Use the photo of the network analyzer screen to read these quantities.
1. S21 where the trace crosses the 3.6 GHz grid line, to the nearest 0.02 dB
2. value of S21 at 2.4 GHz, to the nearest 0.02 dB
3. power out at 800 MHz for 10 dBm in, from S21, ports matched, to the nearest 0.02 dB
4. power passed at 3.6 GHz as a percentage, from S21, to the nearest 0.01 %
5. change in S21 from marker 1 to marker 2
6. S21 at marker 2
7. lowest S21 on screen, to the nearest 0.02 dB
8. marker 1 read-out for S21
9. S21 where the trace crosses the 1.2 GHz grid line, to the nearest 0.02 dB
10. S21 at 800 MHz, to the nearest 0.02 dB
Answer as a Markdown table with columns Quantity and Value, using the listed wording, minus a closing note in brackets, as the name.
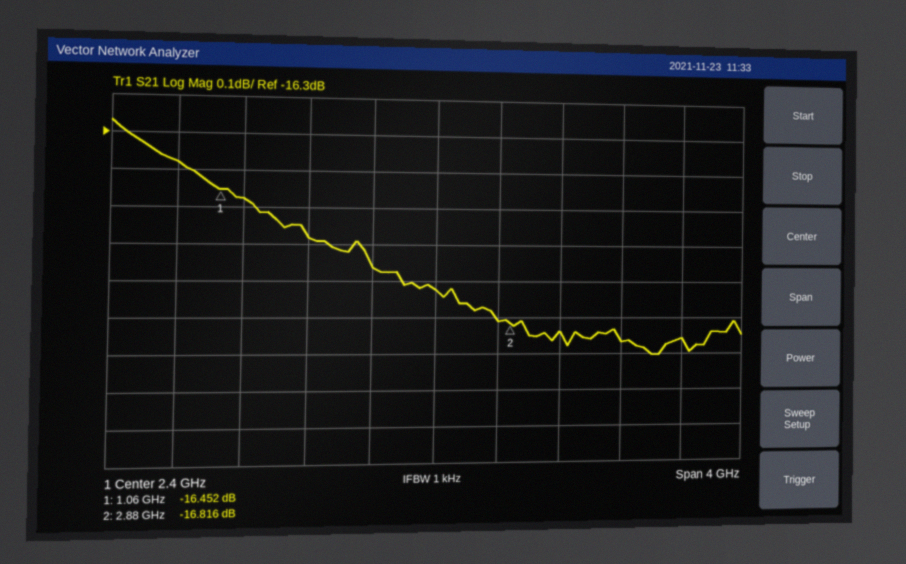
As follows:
| Quantity | Value |
|---|---|
| S21 where the trace crosses the 3.6 GHz grid line, to the nearest 0.02 dB | -16.86 dB |
| value of S21 at 2.4 GHz, to the nearest 0.02 dB | -16.72 dB |
| power out at 800 MHz for 10 dBm in, from S21, ports matched, to the nearest 0.02 dB | -6.38 dBm |
| power passed at 3.6 GHz as a percentage, from S21, to the nearest 0.01 % | 2.06 % |
| change in S21 from marker 1 to marker 2 | -0.364 dB |
| S21 at marker 2 | -16.816 dB |
| lowest S21 on screen, to the nearest 0.02 dB | -16.90 dB |
| marker 1 read-out for S21 | -16.452 dB |
| S21 where the trace crosses the 1.2 GHz grid line, to the nearest 0.02 dB | -16.48 dB |
| S21 at 800 MHz, to the nearest 0.02 dB | -16.38 dB |
